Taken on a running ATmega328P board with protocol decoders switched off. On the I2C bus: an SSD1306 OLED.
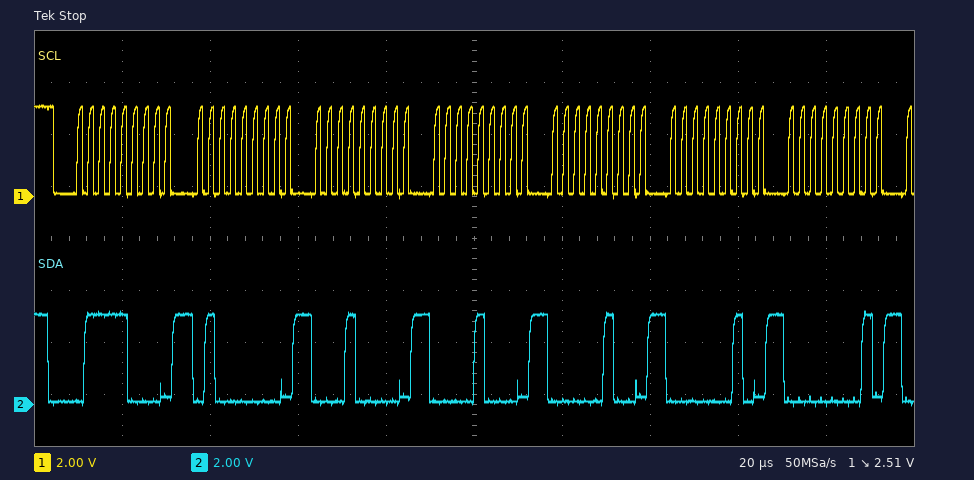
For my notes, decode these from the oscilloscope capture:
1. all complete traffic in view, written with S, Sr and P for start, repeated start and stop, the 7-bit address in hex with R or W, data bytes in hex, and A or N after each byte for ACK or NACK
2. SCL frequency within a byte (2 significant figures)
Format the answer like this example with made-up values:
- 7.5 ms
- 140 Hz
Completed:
- S 3CW A 40 A 10 A 08 A 04 A 02 A 01 A
- 400 kHz
